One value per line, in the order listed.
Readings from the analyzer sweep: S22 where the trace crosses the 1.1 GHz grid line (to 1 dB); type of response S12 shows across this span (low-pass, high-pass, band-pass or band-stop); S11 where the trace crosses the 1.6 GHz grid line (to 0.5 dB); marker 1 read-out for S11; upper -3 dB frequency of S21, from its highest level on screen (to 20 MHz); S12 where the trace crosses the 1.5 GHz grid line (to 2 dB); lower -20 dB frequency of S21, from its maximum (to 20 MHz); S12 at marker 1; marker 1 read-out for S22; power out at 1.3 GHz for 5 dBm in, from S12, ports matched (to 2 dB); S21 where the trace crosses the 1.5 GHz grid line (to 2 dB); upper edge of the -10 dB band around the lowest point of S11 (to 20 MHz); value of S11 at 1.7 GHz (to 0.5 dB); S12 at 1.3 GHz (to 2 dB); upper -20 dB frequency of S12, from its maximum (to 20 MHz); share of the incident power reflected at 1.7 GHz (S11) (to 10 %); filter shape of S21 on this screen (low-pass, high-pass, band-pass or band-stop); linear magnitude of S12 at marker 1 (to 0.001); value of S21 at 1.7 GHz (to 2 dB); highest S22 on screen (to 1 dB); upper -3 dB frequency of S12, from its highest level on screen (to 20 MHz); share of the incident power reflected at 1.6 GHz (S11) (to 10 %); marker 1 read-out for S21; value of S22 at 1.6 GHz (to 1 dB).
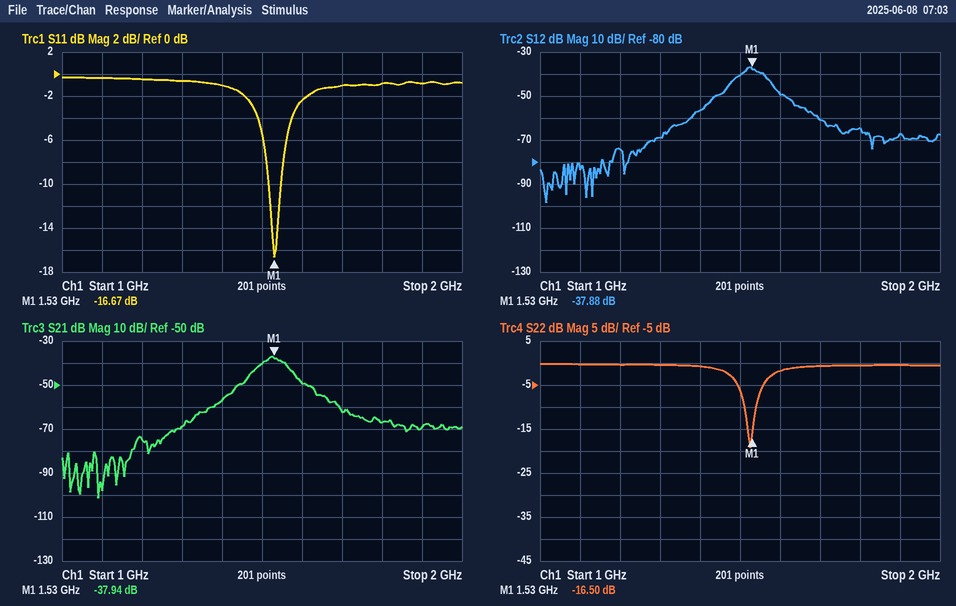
0 dB
band-pass
-2.5 dB
-16.67 dB
1.56 GHz
-40 dB
1.40 GHz
-37.88 dB
-16.50 dB
-64 dBm
-40 dB
1.54 GHz
-1.0 dB
-68 dB
1.66 GHz
80 %
band-pass
0.013
-62 dB
0 dB
1.56 GHz
60 %
-37.94 dB
-2 dB
